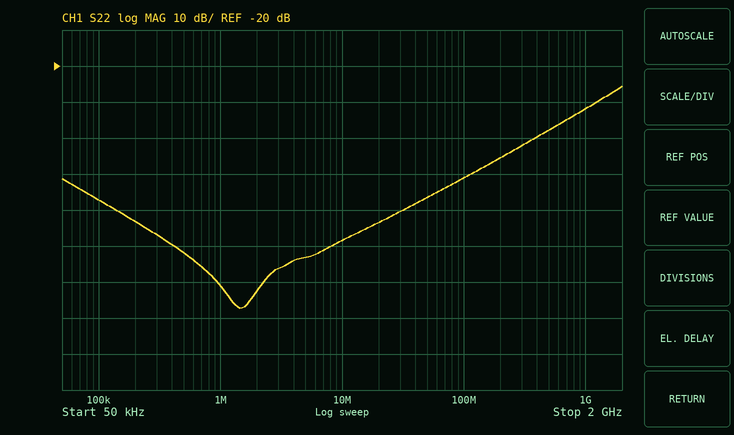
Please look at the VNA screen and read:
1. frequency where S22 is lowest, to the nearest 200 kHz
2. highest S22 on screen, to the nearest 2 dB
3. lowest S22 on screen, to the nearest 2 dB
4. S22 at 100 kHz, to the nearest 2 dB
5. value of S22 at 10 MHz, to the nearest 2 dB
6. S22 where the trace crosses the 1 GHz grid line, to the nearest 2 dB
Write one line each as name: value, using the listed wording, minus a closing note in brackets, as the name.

frequency where S22 is lowest, to the nearest 200 kHz: 1.4 MHz
highest S22 on screen, to the nearest 2 dB: -26 dB
lowest S22 on screen, to the nearest 2 dB: -88 dB
S22 at 100 kHz, to the nearest 2 dB: -58 dB
value of S22 at 10 MHz, to the nearest 2 dB: -68 dB
S22 where the trace crosses the 1 GHz grid line, to the nearest 2 dB: -32 dB
